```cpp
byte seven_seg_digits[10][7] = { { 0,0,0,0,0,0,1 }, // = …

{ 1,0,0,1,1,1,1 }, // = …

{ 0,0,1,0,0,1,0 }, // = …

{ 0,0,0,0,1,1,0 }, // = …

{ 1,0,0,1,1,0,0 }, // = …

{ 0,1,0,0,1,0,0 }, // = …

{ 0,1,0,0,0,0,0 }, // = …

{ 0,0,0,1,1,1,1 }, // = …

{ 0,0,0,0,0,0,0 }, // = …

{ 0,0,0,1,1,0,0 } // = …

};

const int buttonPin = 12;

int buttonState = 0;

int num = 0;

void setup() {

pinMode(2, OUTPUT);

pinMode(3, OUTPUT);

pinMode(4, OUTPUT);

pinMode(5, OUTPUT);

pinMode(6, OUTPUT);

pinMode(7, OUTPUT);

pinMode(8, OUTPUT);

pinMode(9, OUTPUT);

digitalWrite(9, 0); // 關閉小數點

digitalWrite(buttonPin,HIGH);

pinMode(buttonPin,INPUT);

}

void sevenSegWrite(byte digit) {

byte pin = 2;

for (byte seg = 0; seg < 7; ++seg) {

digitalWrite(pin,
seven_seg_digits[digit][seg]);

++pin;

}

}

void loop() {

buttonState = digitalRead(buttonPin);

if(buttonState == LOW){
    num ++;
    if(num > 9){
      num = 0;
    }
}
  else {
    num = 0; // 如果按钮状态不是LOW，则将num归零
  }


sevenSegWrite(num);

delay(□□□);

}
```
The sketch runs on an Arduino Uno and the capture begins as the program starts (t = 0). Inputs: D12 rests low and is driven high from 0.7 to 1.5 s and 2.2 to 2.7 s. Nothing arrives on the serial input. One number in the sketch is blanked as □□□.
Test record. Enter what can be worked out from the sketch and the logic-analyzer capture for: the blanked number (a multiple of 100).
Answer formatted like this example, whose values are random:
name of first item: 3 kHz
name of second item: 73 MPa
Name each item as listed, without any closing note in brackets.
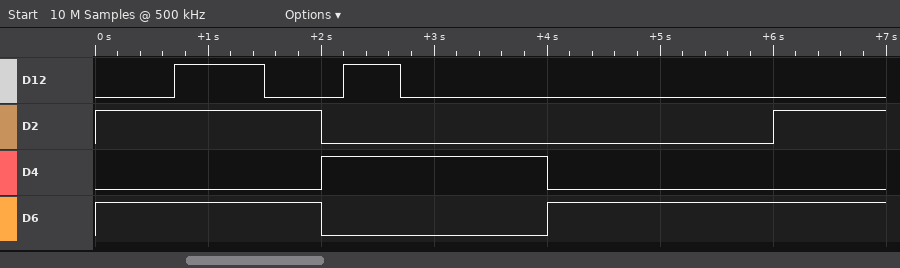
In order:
the blanked number: 2000
